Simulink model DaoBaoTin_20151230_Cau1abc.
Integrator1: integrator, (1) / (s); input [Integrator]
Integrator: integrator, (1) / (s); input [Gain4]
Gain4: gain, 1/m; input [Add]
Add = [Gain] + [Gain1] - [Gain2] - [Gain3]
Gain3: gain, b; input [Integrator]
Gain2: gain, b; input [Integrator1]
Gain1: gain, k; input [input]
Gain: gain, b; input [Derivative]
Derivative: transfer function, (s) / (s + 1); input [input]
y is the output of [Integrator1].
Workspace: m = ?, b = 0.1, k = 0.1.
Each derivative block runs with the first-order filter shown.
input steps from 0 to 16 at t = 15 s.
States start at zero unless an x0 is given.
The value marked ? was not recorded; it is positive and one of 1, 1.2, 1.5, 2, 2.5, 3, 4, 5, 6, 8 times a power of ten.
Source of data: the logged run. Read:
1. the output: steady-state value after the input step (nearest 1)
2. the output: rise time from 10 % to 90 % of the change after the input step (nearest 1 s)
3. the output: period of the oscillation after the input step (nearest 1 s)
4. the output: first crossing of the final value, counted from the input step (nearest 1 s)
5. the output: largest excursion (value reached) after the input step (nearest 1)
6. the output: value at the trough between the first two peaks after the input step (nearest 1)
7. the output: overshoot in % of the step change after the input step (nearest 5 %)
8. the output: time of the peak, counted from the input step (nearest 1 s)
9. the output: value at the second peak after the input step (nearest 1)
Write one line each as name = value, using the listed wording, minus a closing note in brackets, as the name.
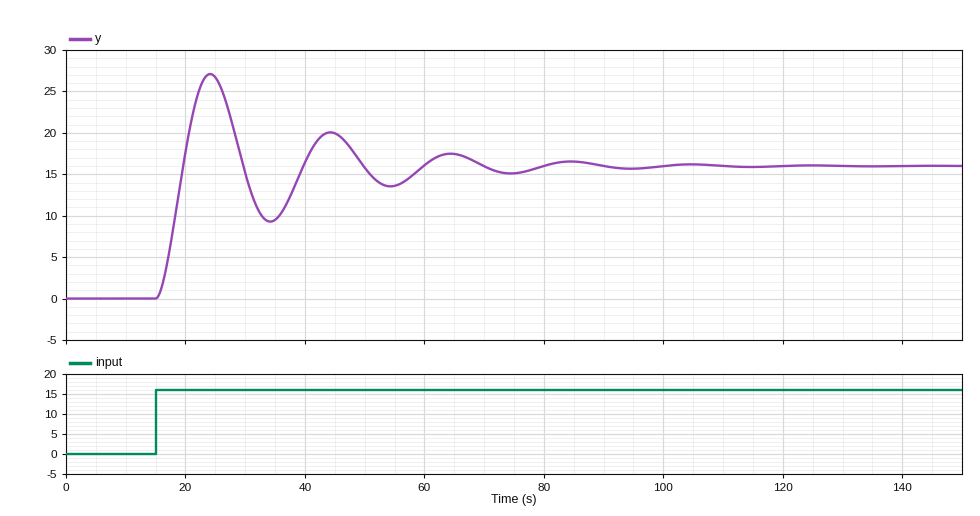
the output: steady-state value after the input step = 16
the output: rise time from 10 % to 90 % of the change after the input step = 3 s
the output: period of the oscillation after the input step = 20 s
the output: first crossing of the final value, counted from the input step = 5 s
the output: largest excursion (value reached) after the input step = 27
the output: value at the trough between the first two peaks after the input step = 9
the output: overshoot in % of the step change after the input step = 70 %
the output: time of the peak, counted from the input step = 9 s
the output: value at the second peak after the input step = 20
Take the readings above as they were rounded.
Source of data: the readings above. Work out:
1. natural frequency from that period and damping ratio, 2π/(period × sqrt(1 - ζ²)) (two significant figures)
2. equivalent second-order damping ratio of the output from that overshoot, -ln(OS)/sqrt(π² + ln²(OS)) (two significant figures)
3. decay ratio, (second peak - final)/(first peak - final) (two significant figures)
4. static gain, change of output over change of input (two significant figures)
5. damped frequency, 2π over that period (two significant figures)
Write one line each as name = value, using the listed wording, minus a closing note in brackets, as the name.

natural frequency from that period and damping ratio, 2π/(period × sqrt(1 - ζ²)) = 0.32 rad/s
equivalent second-order damping ratio of the output from that overshoot, -ln(OS)/sqrt(π² + ln²(OS)) = 0.11
decay ratio, (second peak - final)/(first peak - final) = 0.36
static gain, change of output over change of input = 1.0
damped frequency, 2π over that period = 0.31 rad/s
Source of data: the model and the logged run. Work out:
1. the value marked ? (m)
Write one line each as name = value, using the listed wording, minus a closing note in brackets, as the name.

the value marked ? = 1
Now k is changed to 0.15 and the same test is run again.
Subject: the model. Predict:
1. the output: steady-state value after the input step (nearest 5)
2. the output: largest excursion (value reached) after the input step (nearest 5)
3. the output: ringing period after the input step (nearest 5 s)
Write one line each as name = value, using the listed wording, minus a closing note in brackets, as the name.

the output: steady-state value after the input step = 25
the output: largest excursion (value reached) after the input step = 40
the output: ringing period after the input step = 20 s
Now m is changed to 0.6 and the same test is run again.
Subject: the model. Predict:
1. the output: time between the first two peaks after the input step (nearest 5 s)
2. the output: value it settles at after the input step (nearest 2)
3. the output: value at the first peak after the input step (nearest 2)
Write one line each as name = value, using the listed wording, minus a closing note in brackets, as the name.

the output: time between the first two peaks after the input step = 15 s
the output: value it settles at after the input step = 16
the output: value at the first peak after the input step = 26
